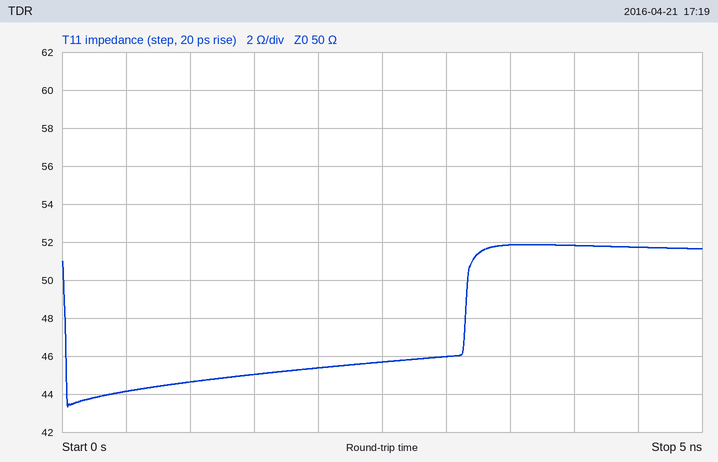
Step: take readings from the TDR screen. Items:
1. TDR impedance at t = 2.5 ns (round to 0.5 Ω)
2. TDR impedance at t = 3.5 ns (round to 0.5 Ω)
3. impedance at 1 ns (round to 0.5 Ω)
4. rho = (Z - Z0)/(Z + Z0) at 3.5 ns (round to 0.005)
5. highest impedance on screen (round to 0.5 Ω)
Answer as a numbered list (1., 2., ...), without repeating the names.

1. 45.5 Ω
2. 52.0 Ω
3. 44.5 Ω
4. +0.020
5. 52.0 Ω
